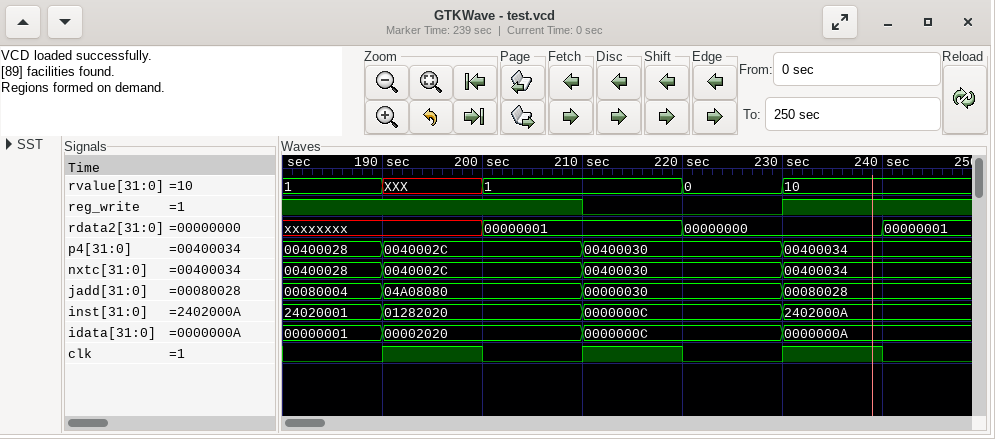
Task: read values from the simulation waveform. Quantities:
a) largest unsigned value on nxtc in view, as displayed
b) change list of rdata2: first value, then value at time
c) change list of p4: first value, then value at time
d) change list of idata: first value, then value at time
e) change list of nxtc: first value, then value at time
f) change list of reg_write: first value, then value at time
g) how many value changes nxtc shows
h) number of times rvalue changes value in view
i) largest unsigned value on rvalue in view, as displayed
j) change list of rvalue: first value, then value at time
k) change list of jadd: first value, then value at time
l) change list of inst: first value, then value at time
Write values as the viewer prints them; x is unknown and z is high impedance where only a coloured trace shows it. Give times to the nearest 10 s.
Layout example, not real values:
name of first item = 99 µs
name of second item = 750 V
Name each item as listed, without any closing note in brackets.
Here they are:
largest unsigned value on nxtc in view, as displayed = 00400034
change list of rdata2: first value, then value at time = xxxxxxxx, 00000001 at 200 s, 00000000 at 220 s, 00000001 at 240 s
change list of p4: first value, then value at time = 00400028, 0040002C at 190 s, 00400030 at 210 s, 00400034 at 230 s
change list of idata: first value, then value at time = 00000001, 00002020 at 190 s, 0000000C at 210 s, 0000000A at 230 s
change list of nxtc: first value, then value at time = 00400028, 0040002C at 190 s, 00400030 at 210 s, 00400034 at 230 s
change list of reg_write: first value, then value at time = 1, 0 at 210 s, 1 at 230 s
how many value changes nxtc shows = 3
number of times rvalue changes value in view = 4
largest unsigned value on rvalue in view, as displayed = 10
change list of rvalue: first value, then value at time = 1, XXX at 190 s, 1 at 200 s, 0 at 220 s, 10 at 230 s
change list of jadd: first value, then value at time = 00080004, 04A08080 at 190 s, 00000030 at 210 s, 00080028 at 230 s
change list of inst: first value, then value at time = 24020001, 01282020 at 190 s, 0000000C at 210 s, 2402000A at 230 s
